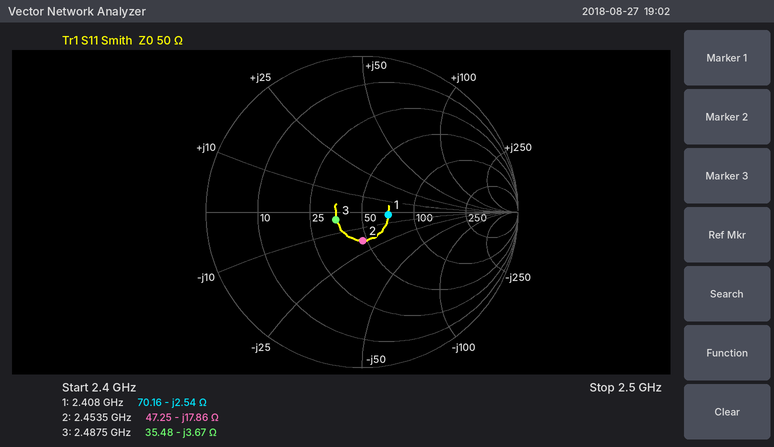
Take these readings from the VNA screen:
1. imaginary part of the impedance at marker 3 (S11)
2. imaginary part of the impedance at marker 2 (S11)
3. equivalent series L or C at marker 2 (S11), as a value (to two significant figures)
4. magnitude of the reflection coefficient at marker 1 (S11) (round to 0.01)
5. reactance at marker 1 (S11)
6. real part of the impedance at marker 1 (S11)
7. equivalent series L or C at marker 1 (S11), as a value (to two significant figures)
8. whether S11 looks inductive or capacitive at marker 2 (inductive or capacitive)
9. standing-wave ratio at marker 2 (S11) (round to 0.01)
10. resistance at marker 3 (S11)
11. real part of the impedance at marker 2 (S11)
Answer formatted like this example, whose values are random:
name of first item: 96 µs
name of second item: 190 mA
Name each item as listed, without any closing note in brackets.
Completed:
imaginary part of the impedance at marker 3: -3.67 Ω
imaginary part of the impedance at marker 2: -17.86 Ω
equivalent series L or C at marker 2 (S11), as a value: 3.6 pF
magnitude of the reflection coefficient at marker 1 (S11): 0.17
reactance at marker 1: -2.54 Ω
real part of the impedance at marker 1: 70.16 Ω
equivalent series L or C at marker 1 (S11), as a value: 26 pF
whether S11 looks inductive or capacitive at marker 2: capacitive
standing-wave ratio at marker 2 (S11): 1.45
resistance at marker 3: 35.48 Ω
real part of the impedance at marker 2: 47.25 Ω
